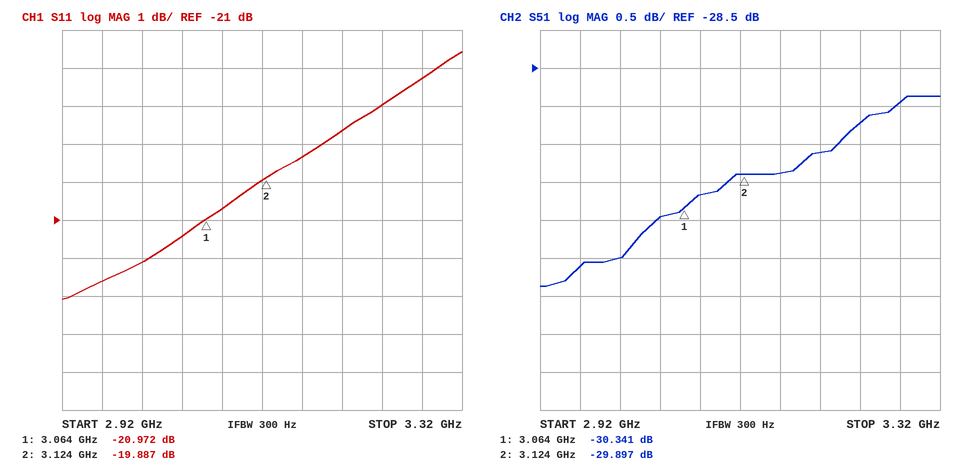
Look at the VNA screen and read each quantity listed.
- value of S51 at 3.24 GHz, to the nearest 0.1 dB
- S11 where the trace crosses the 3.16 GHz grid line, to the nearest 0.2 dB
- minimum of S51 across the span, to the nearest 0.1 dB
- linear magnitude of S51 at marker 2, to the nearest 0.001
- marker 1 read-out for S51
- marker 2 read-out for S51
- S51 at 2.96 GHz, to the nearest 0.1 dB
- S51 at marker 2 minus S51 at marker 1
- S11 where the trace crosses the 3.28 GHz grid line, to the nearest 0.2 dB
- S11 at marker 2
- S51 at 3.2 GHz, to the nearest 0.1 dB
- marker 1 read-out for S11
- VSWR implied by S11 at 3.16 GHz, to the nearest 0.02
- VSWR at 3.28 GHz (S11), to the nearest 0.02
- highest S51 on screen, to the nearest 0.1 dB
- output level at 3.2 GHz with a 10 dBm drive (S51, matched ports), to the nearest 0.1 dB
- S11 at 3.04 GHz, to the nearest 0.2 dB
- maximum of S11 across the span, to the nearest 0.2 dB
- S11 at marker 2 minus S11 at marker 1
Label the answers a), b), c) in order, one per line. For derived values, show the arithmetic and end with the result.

a) -29.2 dB
b) -19.4 dB
c) -31.4 dB
d) 10^(-29.897/20) ≈ 0.032
e) -30.341 dB
f) -29.897 dB
g) -31.1 dB
h) -29.897 − (-30.341) = 0.444 dB
i) -17.2 dB
j) -19.887 dB
k) -29.6 dB
l) -20.972 dB
m) |Γ| = 10^(-19.4/20) = 0.1072; VSWR = (1 + 0.1072)/(1 − 0.1072) ≈ 1.24
n) |Γ| = 10^(-17.2/20) = 0.1380; VSWR = (1 + 0.1380)/(1 − 0.1380) ≈ 1.32
o) -28.9 dB
p) 10 dBm + (-29.6 dB) = -19.6 dBm
q) -21.4 dB
r) -16.6 dB
s) -19.887 − (-20.972) = 1.085 dB
